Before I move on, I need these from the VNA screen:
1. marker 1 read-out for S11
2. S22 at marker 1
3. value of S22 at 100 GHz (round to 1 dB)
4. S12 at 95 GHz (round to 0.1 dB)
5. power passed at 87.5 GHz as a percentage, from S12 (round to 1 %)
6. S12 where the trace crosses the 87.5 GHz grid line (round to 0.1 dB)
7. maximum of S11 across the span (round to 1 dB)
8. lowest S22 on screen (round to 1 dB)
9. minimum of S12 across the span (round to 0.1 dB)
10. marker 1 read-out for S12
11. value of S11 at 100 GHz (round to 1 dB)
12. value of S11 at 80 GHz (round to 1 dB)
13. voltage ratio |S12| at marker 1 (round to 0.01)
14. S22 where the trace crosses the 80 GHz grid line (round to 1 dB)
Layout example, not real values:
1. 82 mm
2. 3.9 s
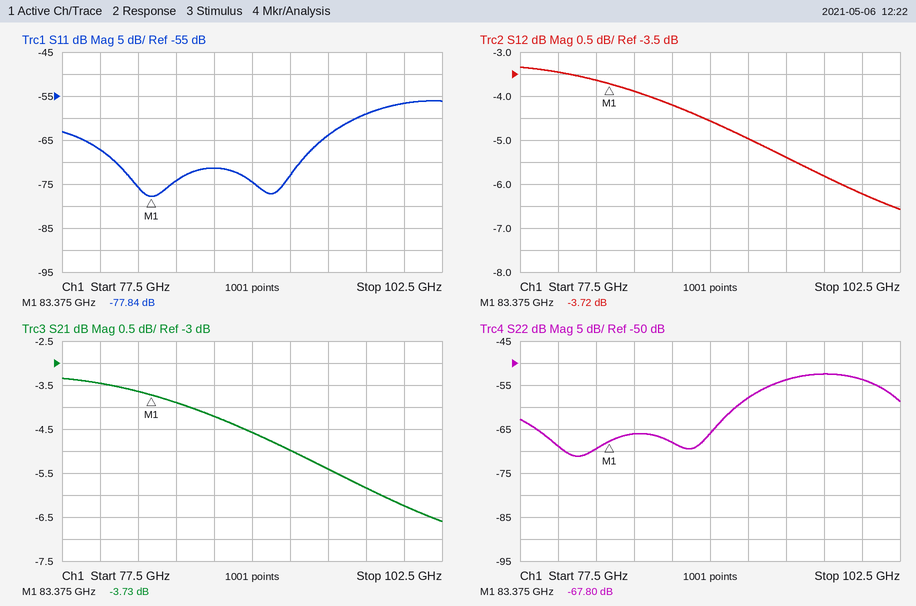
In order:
1. -77.84 dB
2. -67.80 dB
3. -54 dB
4. -5.4 dB
5. 38 %
6. -4.2 dB
7. -56 dB
8. -71 dB
9. -6.6 dB
10. -3.72 dB
11. -57 dB
12. -67 dB
13. 0.65
14. -69 dB
